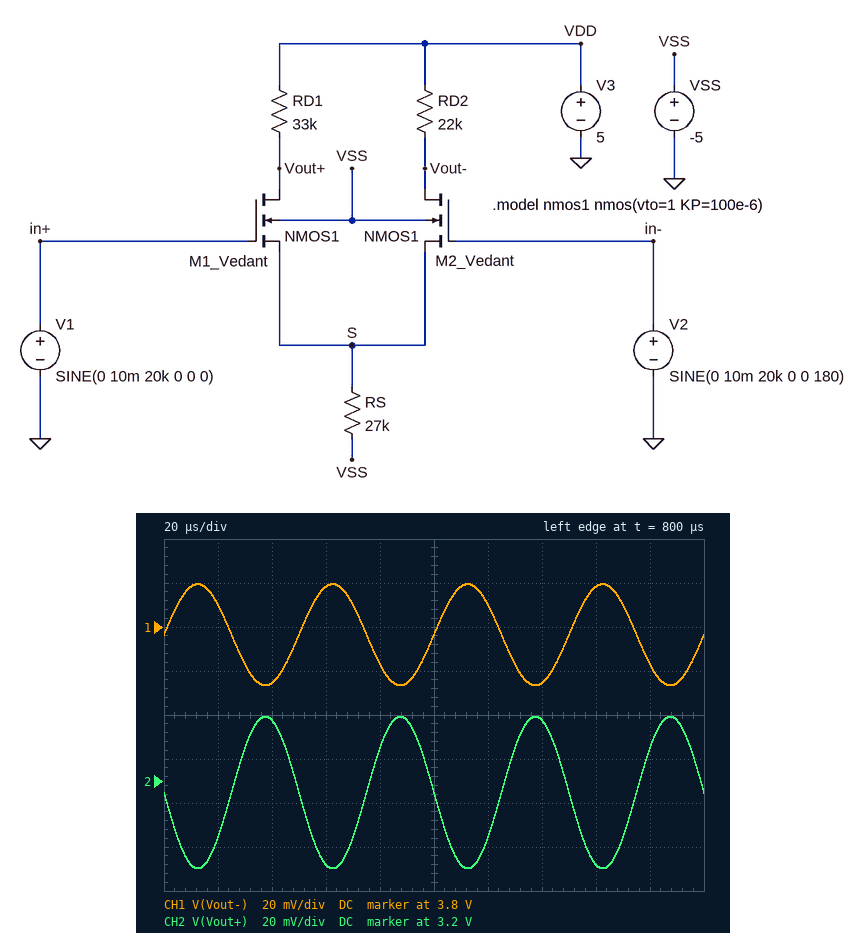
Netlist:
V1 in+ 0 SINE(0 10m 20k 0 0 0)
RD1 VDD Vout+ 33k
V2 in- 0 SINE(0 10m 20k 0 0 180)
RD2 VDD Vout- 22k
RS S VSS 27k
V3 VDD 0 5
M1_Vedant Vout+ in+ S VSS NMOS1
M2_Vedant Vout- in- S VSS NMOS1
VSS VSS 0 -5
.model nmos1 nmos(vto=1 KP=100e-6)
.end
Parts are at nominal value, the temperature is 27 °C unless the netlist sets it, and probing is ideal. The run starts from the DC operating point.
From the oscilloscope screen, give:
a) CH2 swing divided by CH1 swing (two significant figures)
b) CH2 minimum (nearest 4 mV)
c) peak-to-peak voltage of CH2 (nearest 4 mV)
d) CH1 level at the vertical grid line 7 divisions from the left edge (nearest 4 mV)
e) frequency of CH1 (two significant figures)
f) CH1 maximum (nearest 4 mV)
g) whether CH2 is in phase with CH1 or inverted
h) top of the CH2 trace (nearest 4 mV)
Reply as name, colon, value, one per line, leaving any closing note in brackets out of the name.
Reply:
CH2 swing divided by CH1 swing: 1.5
CH2 minimum: 3.160 V
peak-to-peak voltage of CH2: 68 mV
CH1 level at the vertical grid line 7 divisions from the left edge: 3.776 V
frequency of CH1: 20 kHz
CH1 maximum: 3.820 V
whether CH2 is in phase with CH1 or inverted: inverted
top of the CH2 trace: 3.228 V
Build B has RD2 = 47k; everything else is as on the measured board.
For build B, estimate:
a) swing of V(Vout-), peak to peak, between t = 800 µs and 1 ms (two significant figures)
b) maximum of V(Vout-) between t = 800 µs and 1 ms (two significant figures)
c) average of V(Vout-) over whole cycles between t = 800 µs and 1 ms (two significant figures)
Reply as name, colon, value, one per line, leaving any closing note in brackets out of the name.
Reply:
swing of V(Vout-), peak to peak, between t = 800 µs and 1 ms: 98 mV
maximum of V(Vout-) between t = 800 µs and 1 ms: 2.5 V
average of V(Vout-) over whole cycles between t = 800 µs and 1 ms: 2.4 V
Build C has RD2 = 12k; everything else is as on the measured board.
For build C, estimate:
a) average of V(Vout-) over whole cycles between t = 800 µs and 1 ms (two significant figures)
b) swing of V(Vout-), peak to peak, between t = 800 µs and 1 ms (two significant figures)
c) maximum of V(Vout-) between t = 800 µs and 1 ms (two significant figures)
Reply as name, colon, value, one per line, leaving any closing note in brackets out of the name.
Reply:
average of V(Vout-) over whole cycles between t = 800 µs and 1 ms: 4.3 V
swing of V(Vout-), peak to peak, between t = 800 µs and 1 ms: 25 mV
maximum of V(Vout-) between t = 800 µs and 1 ms: 4.4 V
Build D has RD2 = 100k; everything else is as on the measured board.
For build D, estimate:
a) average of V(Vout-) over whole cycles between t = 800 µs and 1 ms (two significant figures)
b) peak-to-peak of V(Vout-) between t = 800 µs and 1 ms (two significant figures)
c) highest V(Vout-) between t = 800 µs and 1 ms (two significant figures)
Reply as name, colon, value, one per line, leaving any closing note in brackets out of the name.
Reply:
average of V(Vout-) over whole cycles between t = 800 µs and 1 ms: -470 mV
peak-to-peak of V(Vout-) between t = 800 µs and 1 ms: 210 mV
highest V(Vout-) between t = 800 µs and 1 ms: -370 mV
